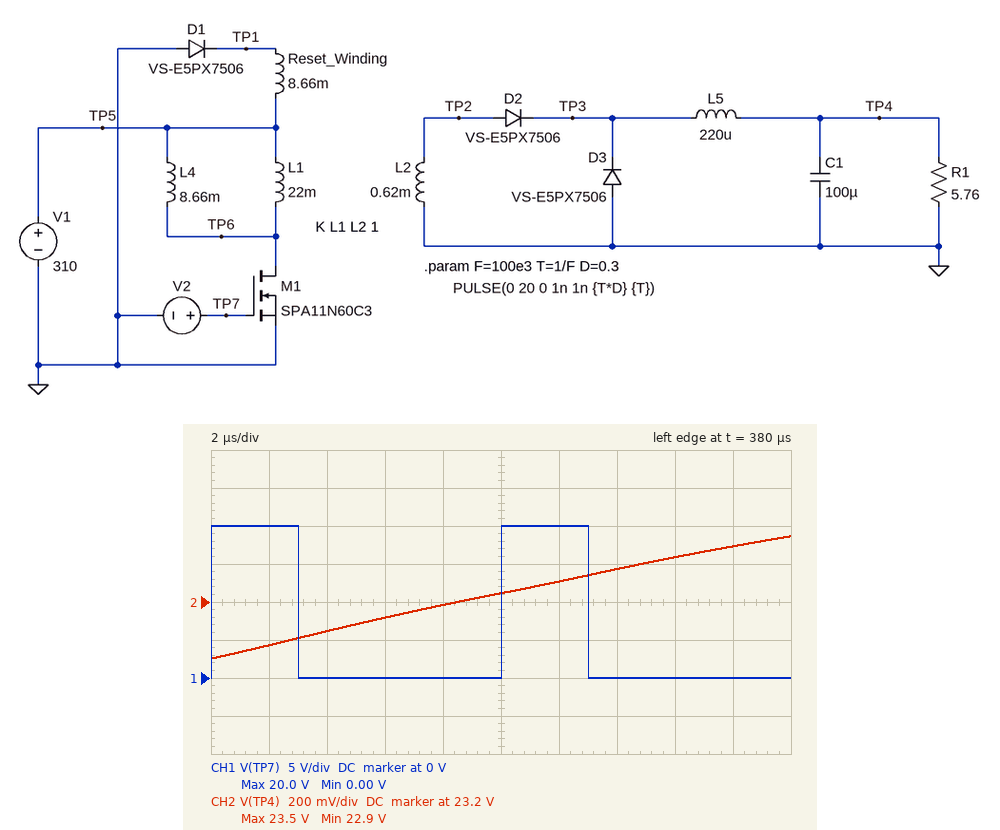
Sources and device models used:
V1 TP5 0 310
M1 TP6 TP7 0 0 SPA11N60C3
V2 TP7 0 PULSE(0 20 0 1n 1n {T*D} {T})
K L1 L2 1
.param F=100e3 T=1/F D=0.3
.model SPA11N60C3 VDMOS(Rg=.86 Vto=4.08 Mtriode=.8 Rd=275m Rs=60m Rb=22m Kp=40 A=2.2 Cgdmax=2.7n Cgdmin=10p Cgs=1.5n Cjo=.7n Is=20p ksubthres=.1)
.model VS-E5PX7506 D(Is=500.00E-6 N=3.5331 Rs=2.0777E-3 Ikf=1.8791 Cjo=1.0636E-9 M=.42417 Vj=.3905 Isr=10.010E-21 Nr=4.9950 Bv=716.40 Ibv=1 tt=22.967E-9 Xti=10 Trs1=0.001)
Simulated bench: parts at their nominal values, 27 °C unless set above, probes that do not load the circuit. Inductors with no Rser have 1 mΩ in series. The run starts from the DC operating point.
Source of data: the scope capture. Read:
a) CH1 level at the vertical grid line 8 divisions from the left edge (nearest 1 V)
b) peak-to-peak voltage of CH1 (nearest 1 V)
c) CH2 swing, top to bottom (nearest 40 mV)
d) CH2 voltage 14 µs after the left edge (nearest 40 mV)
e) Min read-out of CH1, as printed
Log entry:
0 V
20 V
640 mV
23.36 V
0.00 V
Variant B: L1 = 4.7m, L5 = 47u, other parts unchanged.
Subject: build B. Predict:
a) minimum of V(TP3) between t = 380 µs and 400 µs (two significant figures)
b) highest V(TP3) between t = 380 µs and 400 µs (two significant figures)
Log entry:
-970 mV
110 V
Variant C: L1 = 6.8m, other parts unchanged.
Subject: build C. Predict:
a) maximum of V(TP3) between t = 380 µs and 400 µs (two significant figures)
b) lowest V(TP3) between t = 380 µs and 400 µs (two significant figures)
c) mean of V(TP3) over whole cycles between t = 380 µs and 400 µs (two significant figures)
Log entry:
92 V
-1.2 V
27 V
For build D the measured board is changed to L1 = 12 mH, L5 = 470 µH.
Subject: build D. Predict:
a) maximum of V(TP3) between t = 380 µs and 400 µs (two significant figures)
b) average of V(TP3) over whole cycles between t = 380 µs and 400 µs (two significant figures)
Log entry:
69 V
20 V
